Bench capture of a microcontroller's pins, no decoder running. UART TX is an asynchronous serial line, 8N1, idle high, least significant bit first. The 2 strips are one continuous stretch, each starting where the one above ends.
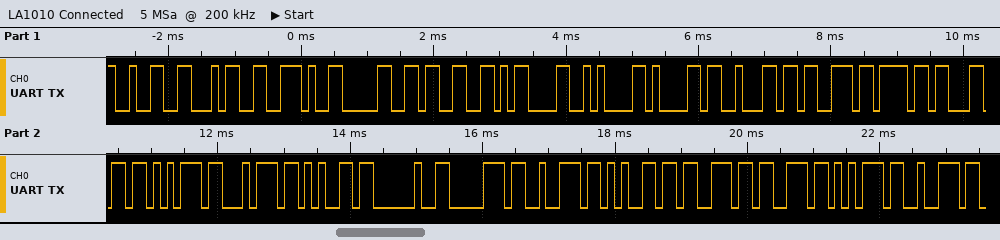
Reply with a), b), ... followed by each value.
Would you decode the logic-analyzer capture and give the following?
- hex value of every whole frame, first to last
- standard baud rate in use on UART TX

a) 32 34 2E 30 33 0D 0A 61 62 73 6F 6C 75 74 65 20 70 72 65 73 73 75 72
b) 9600 baud
